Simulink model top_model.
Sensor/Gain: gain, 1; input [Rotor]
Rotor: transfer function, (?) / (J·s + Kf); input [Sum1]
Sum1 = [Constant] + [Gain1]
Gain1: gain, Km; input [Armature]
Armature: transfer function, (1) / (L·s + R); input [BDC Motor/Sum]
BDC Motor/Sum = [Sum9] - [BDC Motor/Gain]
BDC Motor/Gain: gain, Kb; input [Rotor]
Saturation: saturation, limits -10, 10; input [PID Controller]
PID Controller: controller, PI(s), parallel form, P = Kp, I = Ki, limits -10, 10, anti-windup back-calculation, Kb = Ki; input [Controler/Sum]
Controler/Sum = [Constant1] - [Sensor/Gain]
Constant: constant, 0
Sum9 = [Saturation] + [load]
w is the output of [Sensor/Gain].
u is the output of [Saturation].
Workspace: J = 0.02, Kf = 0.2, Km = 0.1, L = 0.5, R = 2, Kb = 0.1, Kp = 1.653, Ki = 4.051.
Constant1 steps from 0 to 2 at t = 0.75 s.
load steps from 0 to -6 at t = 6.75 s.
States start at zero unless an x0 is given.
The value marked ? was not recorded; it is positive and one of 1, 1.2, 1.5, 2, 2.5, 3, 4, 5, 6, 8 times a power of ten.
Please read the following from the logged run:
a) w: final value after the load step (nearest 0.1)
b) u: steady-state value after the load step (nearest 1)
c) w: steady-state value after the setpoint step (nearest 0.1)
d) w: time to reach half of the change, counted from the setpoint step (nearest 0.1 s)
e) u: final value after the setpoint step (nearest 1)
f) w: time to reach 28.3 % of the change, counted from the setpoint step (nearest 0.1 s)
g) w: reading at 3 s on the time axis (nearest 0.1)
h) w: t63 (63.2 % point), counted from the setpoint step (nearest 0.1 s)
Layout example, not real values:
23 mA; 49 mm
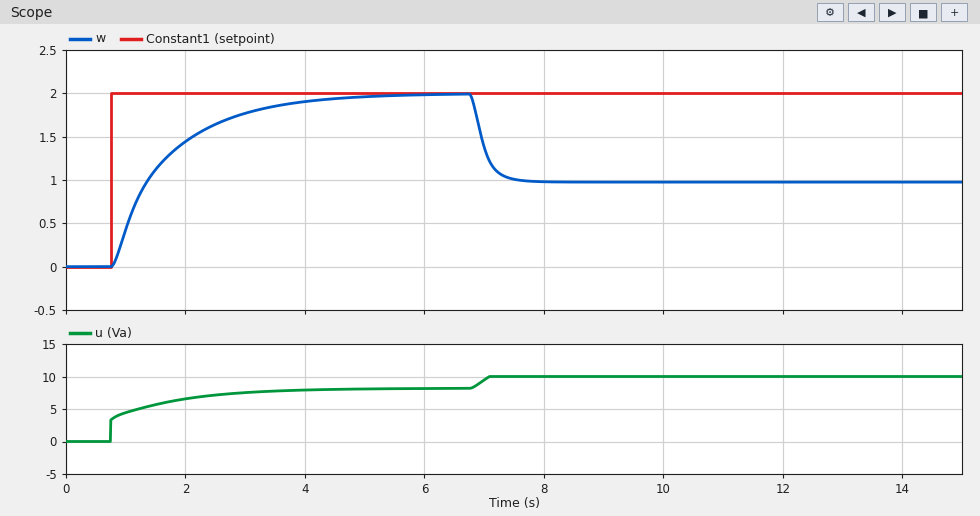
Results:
1.0; 10; 2.0; 0.6 s; 8; 0.3 s; 1.8; 0.9 s
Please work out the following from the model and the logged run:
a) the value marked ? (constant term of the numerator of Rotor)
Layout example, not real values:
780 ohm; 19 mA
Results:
1
